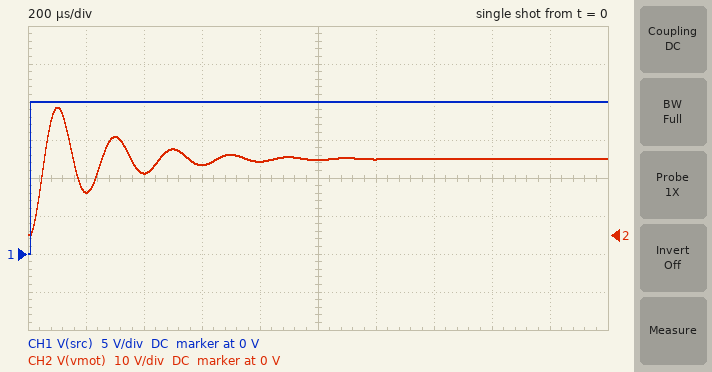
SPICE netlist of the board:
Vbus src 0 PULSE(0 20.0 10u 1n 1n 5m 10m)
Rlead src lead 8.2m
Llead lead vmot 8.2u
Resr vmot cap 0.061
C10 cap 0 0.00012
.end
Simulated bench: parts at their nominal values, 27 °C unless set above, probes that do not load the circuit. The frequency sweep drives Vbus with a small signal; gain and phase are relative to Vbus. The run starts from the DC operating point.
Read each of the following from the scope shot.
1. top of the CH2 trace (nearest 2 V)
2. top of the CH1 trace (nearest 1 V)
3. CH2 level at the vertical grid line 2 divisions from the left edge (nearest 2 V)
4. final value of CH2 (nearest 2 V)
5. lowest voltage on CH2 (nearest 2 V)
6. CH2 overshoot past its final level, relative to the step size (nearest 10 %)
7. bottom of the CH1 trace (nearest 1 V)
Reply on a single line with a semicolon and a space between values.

34 V; 20 V; 16 V; 20 V; 0 V; 70 %; 0 V
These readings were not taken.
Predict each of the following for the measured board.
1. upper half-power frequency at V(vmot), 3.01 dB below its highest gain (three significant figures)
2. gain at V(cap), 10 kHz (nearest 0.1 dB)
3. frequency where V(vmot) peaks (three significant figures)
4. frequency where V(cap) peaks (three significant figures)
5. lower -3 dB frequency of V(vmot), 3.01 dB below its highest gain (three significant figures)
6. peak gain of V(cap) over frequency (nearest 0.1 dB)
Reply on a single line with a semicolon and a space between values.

5.63 kHz; -9.3 dB; 4.99 kHz; 4.98 kHz; 4.26 kHz; 11.6 dB
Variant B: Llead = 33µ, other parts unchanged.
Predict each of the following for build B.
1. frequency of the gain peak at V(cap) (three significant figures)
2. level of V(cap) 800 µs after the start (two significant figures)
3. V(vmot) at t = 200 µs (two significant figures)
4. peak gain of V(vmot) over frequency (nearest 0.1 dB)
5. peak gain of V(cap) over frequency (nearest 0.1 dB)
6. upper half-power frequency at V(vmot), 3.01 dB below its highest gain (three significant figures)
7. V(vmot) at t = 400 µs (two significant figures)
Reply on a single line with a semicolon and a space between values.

2.52 kHz; 11 V; 36 V; 17.7 dB; 17.6 dB; 2.68 kHz; 6.7 V
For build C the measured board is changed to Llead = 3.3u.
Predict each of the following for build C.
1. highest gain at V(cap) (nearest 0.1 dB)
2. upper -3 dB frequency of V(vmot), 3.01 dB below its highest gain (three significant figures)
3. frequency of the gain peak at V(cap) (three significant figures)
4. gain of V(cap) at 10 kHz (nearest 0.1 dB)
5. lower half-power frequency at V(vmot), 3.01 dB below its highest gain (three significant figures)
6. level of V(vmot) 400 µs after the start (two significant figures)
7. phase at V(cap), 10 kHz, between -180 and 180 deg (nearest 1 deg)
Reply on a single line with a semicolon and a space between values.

7.8 dB; 9.26 kHz; 7.64 kHz; 2.3 dB; 5.79 kHz; 20 V; -137 deg
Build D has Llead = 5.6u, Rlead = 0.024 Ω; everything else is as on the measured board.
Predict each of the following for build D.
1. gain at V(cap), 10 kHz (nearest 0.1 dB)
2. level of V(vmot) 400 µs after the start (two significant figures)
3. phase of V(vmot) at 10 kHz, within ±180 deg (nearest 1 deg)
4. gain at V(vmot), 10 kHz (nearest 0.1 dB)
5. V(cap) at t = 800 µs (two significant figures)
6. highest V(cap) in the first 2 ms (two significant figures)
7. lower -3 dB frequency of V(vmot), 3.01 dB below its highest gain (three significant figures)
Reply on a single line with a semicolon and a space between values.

-5.0 dB; 21 V; -134 deg; -4.1 dB; 20 V; 31 V; 4.54 kHz
